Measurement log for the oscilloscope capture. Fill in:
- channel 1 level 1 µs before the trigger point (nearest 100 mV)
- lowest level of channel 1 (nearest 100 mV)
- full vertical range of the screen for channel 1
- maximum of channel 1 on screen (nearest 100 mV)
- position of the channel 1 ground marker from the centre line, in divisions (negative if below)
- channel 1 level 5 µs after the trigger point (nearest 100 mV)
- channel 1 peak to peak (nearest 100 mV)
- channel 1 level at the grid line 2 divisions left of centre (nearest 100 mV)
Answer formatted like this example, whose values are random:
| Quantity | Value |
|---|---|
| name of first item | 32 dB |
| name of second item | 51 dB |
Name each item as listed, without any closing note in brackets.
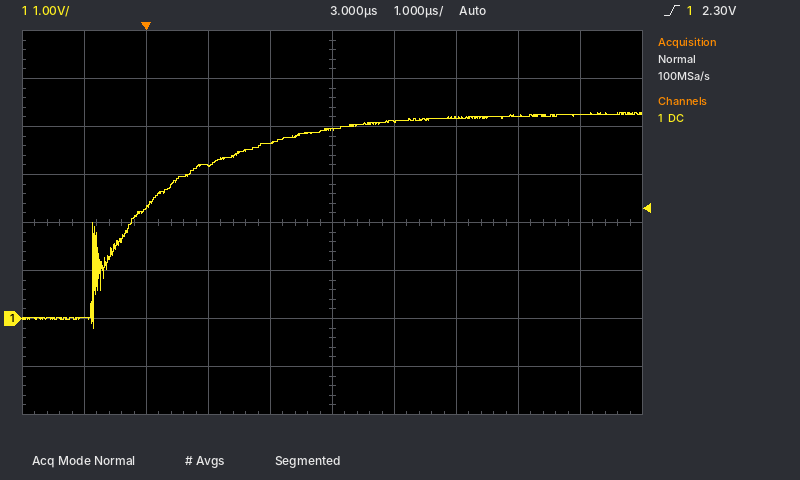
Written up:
| Quantity | Value |
|---|---|
| channel 1 level 1 µs before the trigger point | 0.0 V |
| lowest level of channel 1 | -200 mV |
| full vertical range of the screen for channel 1 | 8 V |
| maximum of channel 1 on screen | 4.3 V |
| position of the channel 1 ground marker from the centre line, in divisions | -2.0 div |
| channel 1 level 5 µs after the trigger point | 4.2 V |
| channel 1 peak to peak | 4.5 V |
| channel 1 level at the grid line 2 divisions left of centre | 3.2 V |
